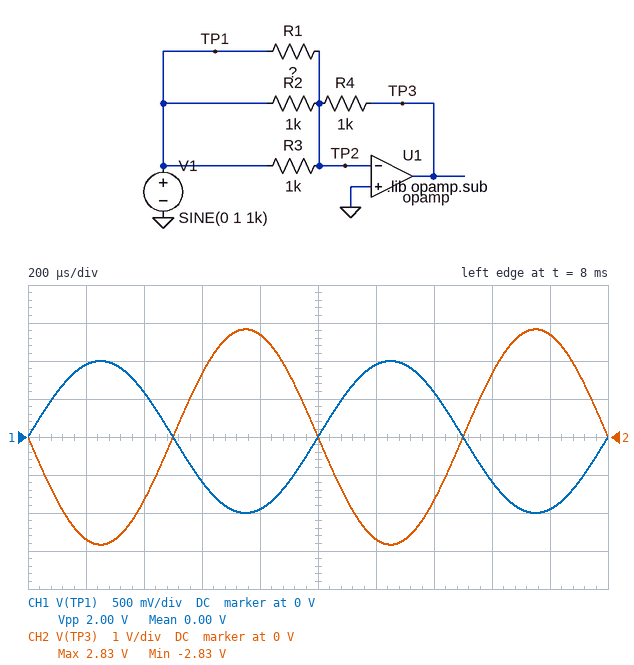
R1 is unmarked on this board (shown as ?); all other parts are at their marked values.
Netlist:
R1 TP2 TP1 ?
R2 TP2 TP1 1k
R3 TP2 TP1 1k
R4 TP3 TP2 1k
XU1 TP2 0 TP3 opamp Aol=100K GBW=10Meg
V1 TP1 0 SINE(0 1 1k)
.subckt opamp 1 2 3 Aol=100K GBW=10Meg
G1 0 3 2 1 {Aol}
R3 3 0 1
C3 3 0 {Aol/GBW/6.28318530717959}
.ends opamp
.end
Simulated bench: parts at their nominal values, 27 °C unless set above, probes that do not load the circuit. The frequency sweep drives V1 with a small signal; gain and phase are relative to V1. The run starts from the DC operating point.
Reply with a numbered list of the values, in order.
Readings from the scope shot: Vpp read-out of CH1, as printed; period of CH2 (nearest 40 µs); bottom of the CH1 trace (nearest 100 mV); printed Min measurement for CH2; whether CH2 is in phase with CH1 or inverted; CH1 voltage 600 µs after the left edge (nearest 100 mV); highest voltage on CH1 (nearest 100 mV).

1. 2.00 V
2. 1.00 ms
3. -1.0 V
4. -2.83 V
5. inverted
6. -600 mV
7. 1.0 V
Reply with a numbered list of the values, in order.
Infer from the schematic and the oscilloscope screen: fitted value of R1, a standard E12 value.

1. 1.2 kΩ
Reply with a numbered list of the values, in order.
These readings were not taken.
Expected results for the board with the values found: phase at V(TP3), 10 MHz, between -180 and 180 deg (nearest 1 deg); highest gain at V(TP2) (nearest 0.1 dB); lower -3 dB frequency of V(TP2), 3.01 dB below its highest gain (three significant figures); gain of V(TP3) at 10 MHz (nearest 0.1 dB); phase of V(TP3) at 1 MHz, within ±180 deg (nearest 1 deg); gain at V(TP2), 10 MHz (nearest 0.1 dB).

1. 105 deg
2. -2.6 dB
3. 2.61 MHz
4. -2.9 dB
5. 159 deg
6. -2.9 dB
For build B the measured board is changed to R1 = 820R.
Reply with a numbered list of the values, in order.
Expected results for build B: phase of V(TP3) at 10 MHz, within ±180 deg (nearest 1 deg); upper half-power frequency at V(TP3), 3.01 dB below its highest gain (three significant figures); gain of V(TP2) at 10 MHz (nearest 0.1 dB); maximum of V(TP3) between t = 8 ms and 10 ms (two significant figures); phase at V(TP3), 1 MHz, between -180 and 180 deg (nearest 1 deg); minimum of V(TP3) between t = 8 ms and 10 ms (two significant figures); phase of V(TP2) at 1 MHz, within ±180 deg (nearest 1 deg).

1. 103 deg
2. 2.37 MHz
3. -2.6 dB
4. 3.2 V
5. 157 deg
6. -3.2 V
7. 67 deg
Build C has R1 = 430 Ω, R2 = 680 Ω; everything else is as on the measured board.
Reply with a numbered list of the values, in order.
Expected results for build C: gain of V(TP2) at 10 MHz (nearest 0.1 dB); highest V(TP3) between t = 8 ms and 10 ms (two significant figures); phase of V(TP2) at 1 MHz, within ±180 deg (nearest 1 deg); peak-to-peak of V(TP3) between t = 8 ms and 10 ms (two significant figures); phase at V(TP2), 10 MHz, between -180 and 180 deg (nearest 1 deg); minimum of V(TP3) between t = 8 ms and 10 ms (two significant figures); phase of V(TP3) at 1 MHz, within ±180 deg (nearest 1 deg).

1. -1.8 dB
2. 4.8 V
3. 60 deg
4. 9.6 V
5. 10 deg
6. -4.8 V
7. 150 deg
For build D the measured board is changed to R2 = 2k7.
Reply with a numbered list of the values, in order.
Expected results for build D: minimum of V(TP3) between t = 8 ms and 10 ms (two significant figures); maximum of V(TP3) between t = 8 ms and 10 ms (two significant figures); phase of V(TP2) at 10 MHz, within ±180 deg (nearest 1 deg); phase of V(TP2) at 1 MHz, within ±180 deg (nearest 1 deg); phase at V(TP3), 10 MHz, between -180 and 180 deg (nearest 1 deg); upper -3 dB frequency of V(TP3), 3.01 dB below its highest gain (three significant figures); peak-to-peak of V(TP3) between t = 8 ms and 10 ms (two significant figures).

1. -2.2 V
2. 2.2 V
3. 17 deg
4. 72 deg
5. 107 deg
6. 3.12 MHz
7. 4.4 V
